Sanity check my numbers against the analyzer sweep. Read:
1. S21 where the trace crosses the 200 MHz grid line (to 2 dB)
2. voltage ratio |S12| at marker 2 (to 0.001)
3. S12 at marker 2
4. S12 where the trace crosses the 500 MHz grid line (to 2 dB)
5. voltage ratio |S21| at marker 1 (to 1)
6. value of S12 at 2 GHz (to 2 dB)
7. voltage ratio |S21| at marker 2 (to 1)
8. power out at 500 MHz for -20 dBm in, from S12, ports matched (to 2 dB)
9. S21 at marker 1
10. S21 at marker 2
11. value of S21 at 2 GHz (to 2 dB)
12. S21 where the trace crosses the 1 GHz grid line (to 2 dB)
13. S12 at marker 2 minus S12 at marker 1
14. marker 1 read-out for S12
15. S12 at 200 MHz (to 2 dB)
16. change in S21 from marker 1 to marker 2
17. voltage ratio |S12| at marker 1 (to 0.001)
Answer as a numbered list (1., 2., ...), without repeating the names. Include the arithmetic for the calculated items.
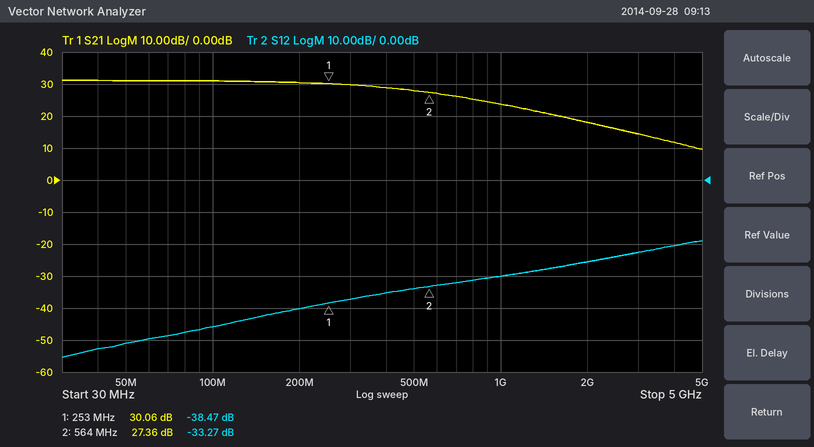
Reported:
1. 30 dB
2. 10^(-33.27/20) ≈ 0.022
3. -33.27 dB
4. -34 dB
5. 10^(30.06/20) ≈ 32
6. -26 dB
7. 10^(27.36/20) ≈ 23
8. -20 dBm + (-34 dB) = -54 dBm
9. 30.06 dB
10. 27.36 dB
11. 18 dB
12. 24 dB
13. -33.27 − (-38.47) = 5.20 dB
14. -38.47 dB
15. -40 dB
16. 27.36 − (30.06) = -2.70 dB
17. 10^(-38.47/20) ≈ 0.012
